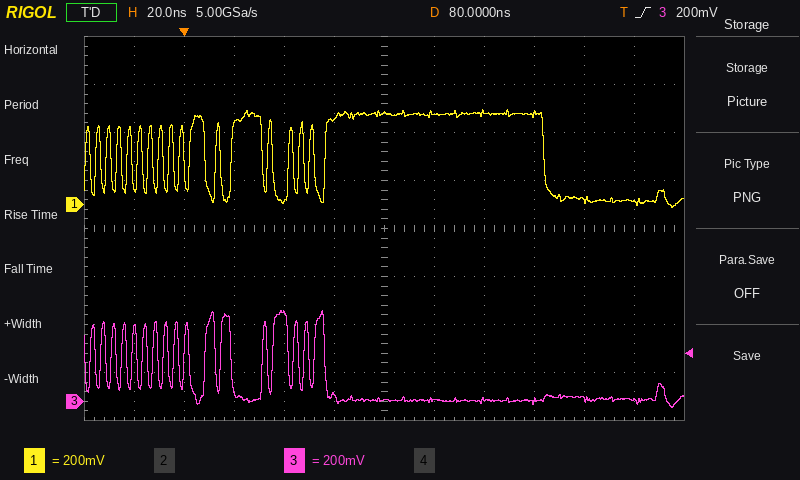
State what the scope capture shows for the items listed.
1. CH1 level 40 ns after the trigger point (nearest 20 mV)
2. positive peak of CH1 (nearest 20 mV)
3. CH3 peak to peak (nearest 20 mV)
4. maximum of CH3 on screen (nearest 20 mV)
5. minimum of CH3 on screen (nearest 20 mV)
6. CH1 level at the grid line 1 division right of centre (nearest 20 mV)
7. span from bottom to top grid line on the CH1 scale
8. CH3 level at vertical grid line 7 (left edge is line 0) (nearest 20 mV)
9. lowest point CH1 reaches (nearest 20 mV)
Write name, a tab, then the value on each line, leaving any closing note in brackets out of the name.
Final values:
CH1 level 40 ns after the trigger point	20 mV
positive peak of CH1	400 mV
CH3 peak to peak	400 mV
maximum of CH3 on screen	380 mV
minimum of CH3 on screen	-20 mV
CH1 level at the grid line 1 division right of centre	380 mV
span from bottom to top grid line on the CH1 scale	1.6 V
CH3 level at vertical grid line 7 (left edge is line 0)	0 mV
lowest point CH1 reaches	-20 mV
